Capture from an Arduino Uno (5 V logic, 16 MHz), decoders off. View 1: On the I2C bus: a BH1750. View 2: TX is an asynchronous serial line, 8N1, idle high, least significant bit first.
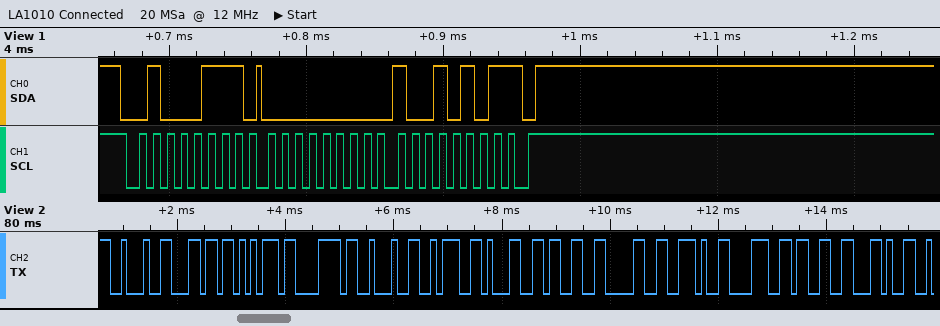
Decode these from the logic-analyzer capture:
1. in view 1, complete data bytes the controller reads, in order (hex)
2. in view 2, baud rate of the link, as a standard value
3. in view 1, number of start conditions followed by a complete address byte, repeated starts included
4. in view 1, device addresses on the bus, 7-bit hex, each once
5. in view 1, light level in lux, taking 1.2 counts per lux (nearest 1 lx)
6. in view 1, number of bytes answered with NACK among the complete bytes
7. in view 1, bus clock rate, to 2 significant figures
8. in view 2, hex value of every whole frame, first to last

00 95
9600 baud
1
0x23
124 lx
1
100 kHz
22 6C 75 78 22 3A 31 33 30 2E 38 33 2C
